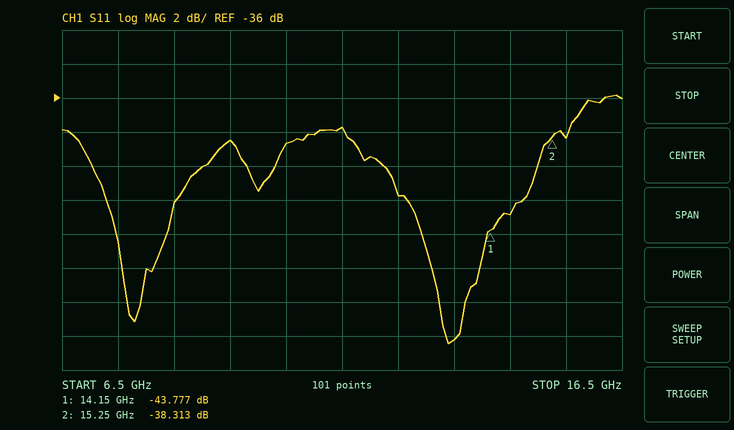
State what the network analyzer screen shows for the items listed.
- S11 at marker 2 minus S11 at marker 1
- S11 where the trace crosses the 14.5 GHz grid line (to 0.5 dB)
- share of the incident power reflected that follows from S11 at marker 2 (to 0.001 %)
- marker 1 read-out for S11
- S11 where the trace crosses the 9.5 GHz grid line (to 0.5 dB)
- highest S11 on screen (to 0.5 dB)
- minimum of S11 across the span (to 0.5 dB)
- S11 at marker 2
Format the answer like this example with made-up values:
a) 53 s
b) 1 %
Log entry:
a) 5.464 dB
b) -43.0 dB
c) 0.015 %
d) -43.777 dB
e) -38.5 dB
f) -36.0 dB
g) -50.5 dB
h) -38.313 dB
